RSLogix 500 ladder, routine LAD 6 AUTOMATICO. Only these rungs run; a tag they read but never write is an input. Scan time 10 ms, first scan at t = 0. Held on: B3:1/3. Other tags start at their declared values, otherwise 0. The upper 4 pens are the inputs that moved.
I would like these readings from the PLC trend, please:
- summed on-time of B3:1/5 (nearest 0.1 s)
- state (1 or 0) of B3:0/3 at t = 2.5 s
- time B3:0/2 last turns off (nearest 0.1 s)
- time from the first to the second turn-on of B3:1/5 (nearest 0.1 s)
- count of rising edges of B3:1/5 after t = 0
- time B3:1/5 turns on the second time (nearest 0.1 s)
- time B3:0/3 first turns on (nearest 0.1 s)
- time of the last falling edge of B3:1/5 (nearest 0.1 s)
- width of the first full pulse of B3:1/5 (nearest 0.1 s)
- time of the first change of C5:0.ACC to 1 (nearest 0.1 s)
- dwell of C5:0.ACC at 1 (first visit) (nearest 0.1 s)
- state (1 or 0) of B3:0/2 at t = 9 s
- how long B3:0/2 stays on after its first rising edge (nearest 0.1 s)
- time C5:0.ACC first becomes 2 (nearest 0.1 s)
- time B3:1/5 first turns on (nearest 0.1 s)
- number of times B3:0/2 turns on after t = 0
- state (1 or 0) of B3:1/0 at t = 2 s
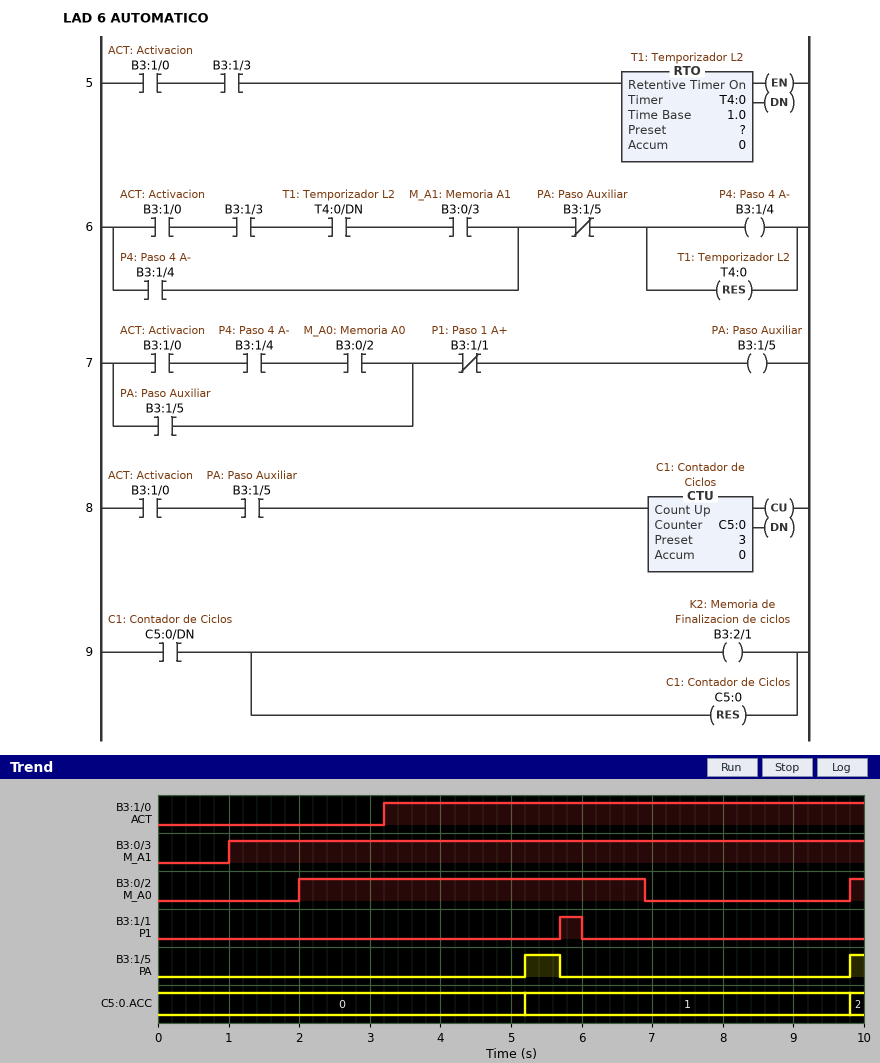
0.7 s
1
6.9 s
4.6 s
2
9.8 s
1.0 s
5.7 s
0.5 s
5.2 s
4.6 s
0
4.9 s
9.8 s
5.2 s
2
0
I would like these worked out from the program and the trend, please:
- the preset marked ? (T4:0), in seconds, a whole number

2 s
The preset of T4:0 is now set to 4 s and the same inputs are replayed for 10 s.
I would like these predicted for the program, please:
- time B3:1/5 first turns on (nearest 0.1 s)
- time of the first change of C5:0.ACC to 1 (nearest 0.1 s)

9.8 s
9.8 s
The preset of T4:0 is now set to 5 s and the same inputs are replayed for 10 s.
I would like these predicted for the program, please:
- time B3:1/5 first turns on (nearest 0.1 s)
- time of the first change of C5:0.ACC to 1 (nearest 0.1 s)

9.8 s
9.8 s
